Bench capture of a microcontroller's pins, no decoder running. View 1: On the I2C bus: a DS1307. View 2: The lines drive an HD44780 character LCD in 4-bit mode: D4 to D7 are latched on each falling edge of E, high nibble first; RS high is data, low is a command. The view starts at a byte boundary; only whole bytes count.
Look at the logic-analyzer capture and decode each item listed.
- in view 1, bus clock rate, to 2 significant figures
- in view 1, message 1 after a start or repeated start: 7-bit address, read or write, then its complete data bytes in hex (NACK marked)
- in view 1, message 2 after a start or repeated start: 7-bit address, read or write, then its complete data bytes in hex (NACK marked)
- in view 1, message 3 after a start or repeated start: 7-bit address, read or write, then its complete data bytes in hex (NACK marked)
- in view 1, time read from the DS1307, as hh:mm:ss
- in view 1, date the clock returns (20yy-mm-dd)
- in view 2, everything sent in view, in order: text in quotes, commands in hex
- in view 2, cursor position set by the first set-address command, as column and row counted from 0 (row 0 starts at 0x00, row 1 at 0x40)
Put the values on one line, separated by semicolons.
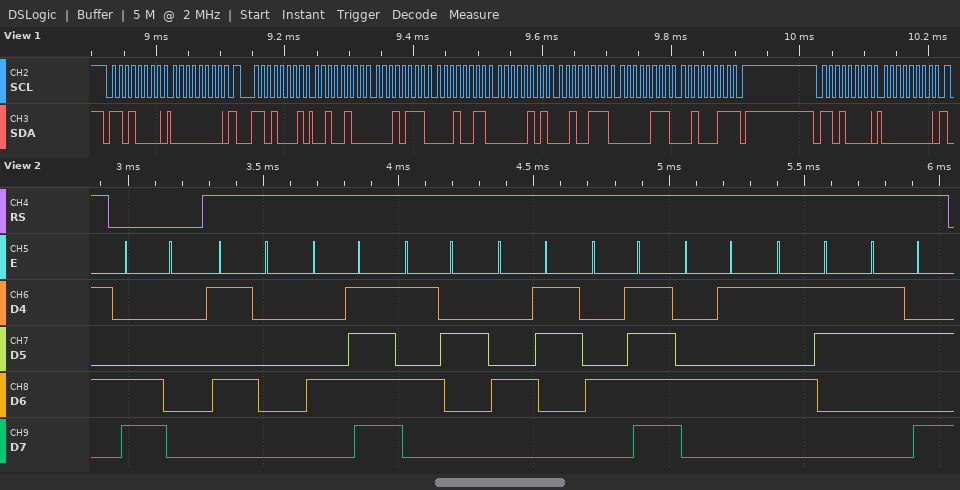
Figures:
100 kHz; 0x68 write: 00; 0x68 read: 24 17 13 05 27 07 23 NACK; 0x68 write: 00; 13:17:24; 2023-07-27; 0xC0 "PORCOES:"; column 0, row 1
